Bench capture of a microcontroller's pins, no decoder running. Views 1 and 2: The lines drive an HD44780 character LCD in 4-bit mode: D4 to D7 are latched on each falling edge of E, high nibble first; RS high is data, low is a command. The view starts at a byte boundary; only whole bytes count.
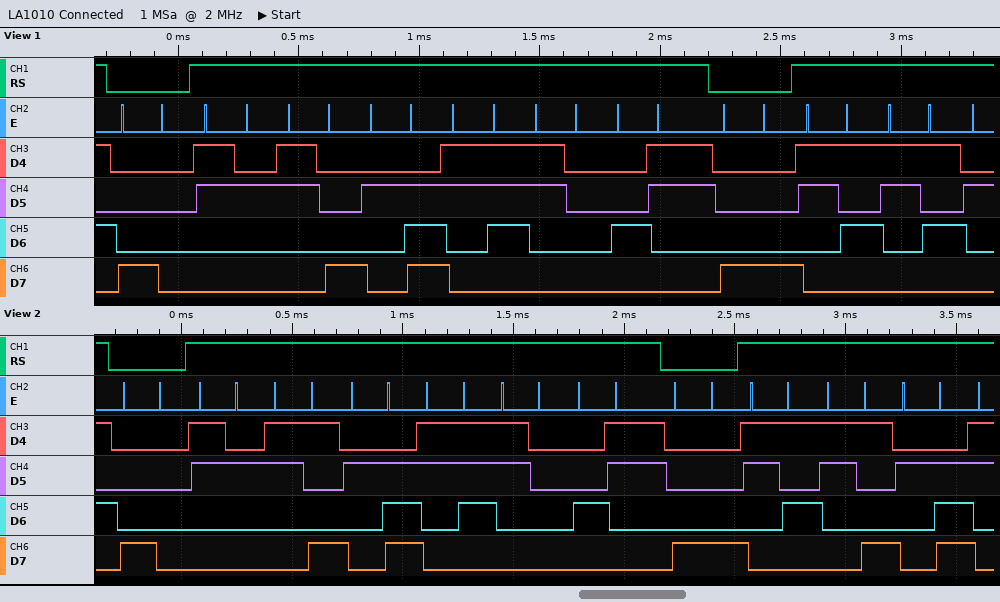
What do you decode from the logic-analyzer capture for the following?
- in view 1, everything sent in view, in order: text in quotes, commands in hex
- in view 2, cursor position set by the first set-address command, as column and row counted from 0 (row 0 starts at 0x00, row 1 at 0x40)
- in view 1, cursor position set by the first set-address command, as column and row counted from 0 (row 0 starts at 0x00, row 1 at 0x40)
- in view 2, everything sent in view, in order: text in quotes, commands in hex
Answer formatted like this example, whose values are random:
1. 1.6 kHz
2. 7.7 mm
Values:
1. 0x80 "28.70C" 0x88 "55"
2. column 0, row 0
3. column 0, row 0
4. 0x80 "29.70C" 0x88 "59."
